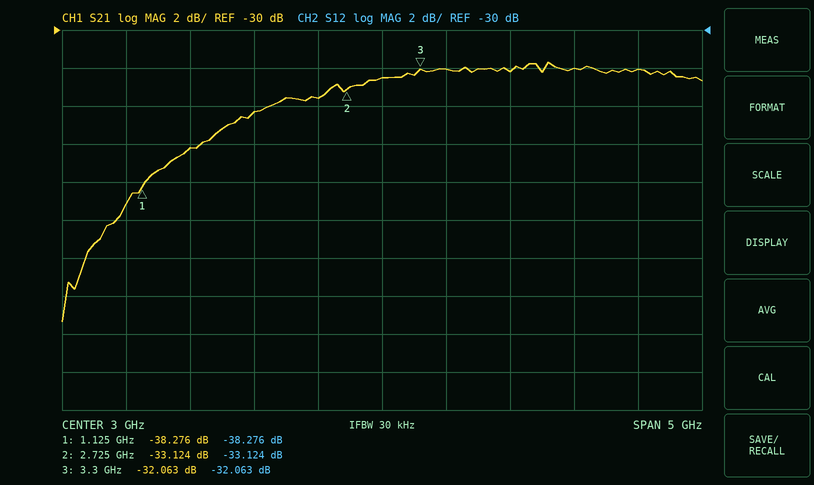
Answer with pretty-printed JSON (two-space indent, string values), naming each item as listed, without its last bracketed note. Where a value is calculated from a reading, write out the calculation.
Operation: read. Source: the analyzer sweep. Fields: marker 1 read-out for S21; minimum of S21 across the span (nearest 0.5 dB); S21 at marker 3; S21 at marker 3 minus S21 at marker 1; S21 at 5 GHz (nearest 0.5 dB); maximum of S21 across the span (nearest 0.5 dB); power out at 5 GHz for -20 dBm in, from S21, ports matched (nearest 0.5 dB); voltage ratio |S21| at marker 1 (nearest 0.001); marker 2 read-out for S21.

{
  "marker 1 read-out for S21": "-38.276 dB",
  "minimum of S21 across the span": "-45.5 dB",
  "S21 at marker 3": "-32.063 dB",
  "S21 at marker 3 minus S21 at marker 1": "-32.063 − (-38.276) = 6.213 dB",
  "S21 at 5 GHz": "-32.0 dB",
  "maximum of S21 across the span": "-31.5 dB",
  "power out at 5 GHz for -20 dBm in, from S21, ports matched": "-20 dBm + (-32.0 dB) = -52.0 dBm",
  "voltage ratio |S21| at marker 1": "10^(-38.276/20) ≈ 0.012",
  "marker 2 read-out for S21": "-33.124 dB"
}
